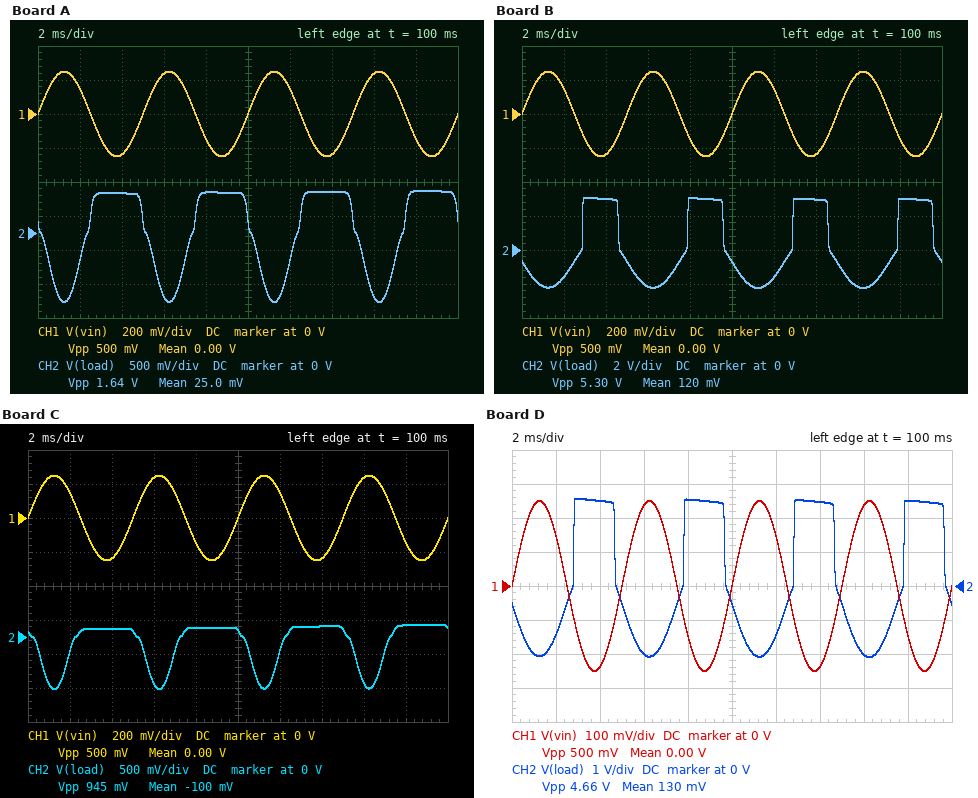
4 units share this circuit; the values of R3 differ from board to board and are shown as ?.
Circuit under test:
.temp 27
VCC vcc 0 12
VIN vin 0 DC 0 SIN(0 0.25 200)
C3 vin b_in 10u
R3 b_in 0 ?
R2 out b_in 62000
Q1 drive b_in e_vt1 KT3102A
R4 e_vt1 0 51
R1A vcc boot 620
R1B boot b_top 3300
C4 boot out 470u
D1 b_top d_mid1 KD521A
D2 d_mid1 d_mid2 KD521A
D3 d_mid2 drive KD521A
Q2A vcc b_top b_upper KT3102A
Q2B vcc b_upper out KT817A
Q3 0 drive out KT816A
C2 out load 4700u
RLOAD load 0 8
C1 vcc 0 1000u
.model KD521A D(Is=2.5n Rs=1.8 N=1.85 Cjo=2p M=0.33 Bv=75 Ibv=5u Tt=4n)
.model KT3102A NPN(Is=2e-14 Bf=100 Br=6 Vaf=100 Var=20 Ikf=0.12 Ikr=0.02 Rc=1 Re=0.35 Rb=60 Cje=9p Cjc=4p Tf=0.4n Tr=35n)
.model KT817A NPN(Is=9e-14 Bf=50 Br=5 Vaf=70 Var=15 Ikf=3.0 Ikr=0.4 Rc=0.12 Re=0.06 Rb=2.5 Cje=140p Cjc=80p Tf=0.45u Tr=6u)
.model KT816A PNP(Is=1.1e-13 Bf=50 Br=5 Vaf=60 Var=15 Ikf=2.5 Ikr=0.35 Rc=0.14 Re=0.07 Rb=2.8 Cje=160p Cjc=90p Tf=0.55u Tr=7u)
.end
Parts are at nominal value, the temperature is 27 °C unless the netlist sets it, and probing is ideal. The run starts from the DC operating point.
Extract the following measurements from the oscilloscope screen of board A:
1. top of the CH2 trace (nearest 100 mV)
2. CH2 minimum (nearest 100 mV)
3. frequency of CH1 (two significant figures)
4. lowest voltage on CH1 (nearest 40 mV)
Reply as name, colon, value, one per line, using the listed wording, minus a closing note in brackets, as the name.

top of the CH2 trace: 600 mV
CH2 minimum: -1.0 V
frequency of CH1: 200 Hz
lowest voltage on CH1: -240 mV
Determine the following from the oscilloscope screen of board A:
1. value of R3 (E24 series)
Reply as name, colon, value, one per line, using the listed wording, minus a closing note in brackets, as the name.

value of R3: 3.6 kΩ
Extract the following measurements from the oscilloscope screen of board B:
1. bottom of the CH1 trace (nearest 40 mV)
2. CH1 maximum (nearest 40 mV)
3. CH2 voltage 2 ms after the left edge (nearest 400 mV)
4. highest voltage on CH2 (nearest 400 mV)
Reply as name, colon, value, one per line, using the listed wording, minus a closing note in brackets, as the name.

bottom of the CH1 trace: -240 mV
CH1 maximum: 240 mV
CH2 voltage 2 ms after the left edge: -1.6 V
highest voltage on CH2: 3.2 V
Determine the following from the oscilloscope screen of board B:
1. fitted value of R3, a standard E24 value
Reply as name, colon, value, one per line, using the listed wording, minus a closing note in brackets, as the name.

fitted value of R3, a standard E24 value: 9.1 kΩ
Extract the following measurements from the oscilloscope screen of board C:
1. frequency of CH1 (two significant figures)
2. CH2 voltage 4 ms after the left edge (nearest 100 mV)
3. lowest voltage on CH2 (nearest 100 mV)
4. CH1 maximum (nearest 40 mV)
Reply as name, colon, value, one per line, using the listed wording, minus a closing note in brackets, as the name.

frequency of CH1: 200 Hz
CH2 voltage 4 ms after the left edge: 100 mV
lowest voltage on CH2: -800 mV
CH1 maximum: 240 mV
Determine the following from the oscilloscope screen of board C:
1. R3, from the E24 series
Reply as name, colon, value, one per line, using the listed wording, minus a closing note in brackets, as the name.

R3, from the E24 series: 3.3 kΩ
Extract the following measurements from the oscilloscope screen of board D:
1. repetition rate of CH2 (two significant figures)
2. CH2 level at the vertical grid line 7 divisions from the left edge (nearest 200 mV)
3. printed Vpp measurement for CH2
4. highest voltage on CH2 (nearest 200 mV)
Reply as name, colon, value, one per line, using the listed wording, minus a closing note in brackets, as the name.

repetition rate of CH2: 200 Hz
CH2 level at the vertical grid line 7 divisions from the left edge: 2.4 V
printed Vpp measurement for CH2: 4.66 V
highest voltage on CH2: 2.6 V
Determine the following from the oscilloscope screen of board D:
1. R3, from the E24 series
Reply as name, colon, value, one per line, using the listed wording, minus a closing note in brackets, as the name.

R3, from the E24 series: 7.5 kΩ
